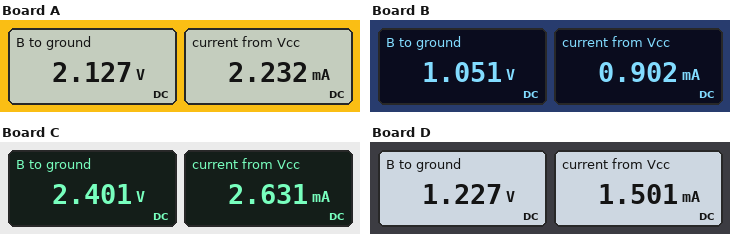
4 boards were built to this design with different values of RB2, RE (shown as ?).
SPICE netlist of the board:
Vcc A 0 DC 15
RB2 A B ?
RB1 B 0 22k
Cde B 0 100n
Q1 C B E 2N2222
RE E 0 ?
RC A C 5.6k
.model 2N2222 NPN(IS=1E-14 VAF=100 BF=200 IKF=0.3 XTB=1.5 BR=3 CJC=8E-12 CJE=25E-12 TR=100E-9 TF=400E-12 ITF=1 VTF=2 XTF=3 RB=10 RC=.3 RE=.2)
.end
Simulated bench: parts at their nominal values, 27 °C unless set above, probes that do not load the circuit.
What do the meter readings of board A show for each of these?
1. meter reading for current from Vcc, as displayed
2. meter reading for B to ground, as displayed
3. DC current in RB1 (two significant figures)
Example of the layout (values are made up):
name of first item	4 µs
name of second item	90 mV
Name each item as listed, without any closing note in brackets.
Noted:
meter reading for current from Vcc, as displayed	2.232 mA
meter reading for B to ground, as displayed	2.127 V
DC current in RB1	97 µA
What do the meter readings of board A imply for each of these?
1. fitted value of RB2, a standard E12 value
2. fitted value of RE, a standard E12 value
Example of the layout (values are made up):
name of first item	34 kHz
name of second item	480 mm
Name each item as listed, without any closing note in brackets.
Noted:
fitted value of RB2, a standard E12 value	120 kΩ
fitted value of RE, a standard E12 value	680 Ω
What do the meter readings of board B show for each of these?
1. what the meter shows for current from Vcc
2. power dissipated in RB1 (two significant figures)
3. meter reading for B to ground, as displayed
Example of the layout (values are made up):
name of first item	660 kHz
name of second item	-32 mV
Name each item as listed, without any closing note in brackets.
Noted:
what the meter shows for current from Vcc	0.902 mA
power dissipated in RB1	50 µW
meter reading for B to ground, as displayed	1.051 V
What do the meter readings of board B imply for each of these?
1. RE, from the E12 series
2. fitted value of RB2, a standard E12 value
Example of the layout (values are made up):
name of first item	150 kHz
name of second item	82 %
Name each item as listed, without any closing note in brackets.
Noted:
RE, from the E12 series	470 Ω
fitted value of RB2, a standard E12 value	270 kΩ
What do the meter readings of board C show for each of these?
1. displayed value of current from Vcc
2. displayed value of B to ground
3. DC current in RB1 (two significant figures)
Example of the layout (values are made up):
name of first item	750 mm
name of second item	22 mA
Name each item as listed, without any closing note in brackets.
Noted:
displayed value of current from Vcc	2.631 mA
displayed value of B to ground	2.401 V
DC current in RB1	110 µA
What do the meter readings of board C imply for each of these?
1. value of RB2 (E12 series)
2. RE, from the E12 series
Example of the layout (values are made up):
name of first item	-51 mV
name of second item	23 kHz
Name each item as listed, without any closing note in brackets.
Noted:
value of RB2	47 kΩ
RE, from the E12 series	680 Ω
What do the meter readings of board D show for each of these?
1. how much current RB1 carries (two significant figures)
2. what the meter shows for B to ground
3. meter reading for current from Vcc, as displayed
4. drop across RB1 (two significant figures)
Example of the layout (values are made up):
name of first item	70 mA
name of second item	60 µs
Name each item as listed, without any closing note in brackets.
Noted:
how much current RB1 carries	56 µA
what the meter shows for B to ground	1.227 V
meter reading for current from Vcc, as displayed	1.501 mA
drop across RB1	1.2 V
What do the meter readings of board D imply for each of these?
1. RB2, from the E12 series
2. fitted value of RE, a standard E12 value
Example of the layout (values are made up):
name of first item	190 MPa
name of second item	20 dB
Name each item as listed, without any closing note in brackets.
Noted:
RB2, from the E12 series	220 kΩ
fitted value of RE, a standard E12 value	390 Ω
